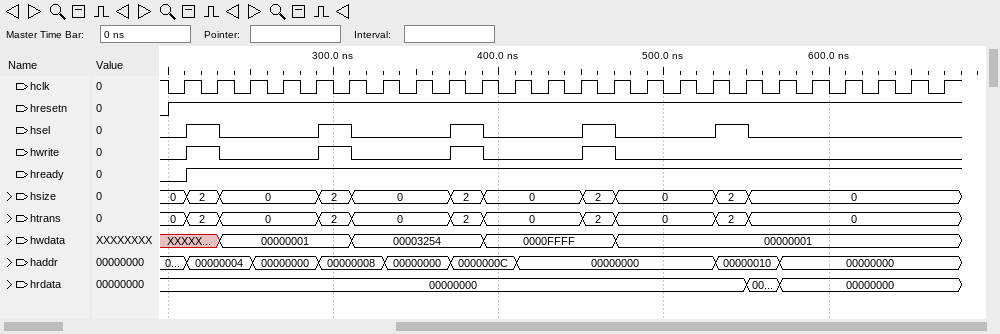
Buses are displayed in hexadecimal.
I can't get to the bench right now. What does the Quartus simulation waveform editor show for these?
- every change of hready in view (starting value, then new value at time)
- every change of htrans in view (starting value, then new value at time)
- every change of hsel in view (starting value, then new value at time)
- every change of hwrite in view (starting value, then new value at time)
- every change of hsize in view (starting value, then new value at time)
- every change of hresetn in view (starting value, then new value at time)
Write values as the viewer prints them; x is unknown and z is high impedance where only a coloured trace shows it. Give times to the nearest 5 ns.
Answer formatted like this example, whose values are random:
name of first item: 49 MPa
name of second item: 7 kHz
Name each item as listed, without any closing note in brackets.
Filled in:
every change of hready in view: 0, 1 at 210 ns
every change of htrans in view: 0, 2 at 210 ns, 0 at 230 ns, 2 at 290 ns, 0 at 310 ns, 2 at 370 ns, 0 at 390 ns, 2 at 450 ns, 0 at 470 ns, 2 at 530 ns, 0 at 550 ns
every change of hsel in view: 0, 1 at 210 ns, 0 at 230 ns, 1 at 290 ns, 0 at 310 ns, 1 at 370 ns, 0 at 390 ns, 1 at 450 ns, 0 at 470 ns, 1 at 530 ns, 0 at 550 ns
every change of hwrite in view: 0, 1 at 210 ns, 0 at 230 ns, 1 at 290 ns, 0 at 310 ns, 1 at 370 ns, 0 at 390 ns, 1 at 450 ns, 0 at 470 ns
every change of hsize in view: 0, 2 at 210 ns, 0 at 230 ns, 2 at 290 ns, 0 at 310 ns, 2 at 370 ns, 0 at 390 ns, 2 at 450 ns, 0 at 470 ns, 2 at 530 ns, 0 at 550 ns
every change of hresetn in view: 0, 1 at 200 ns
